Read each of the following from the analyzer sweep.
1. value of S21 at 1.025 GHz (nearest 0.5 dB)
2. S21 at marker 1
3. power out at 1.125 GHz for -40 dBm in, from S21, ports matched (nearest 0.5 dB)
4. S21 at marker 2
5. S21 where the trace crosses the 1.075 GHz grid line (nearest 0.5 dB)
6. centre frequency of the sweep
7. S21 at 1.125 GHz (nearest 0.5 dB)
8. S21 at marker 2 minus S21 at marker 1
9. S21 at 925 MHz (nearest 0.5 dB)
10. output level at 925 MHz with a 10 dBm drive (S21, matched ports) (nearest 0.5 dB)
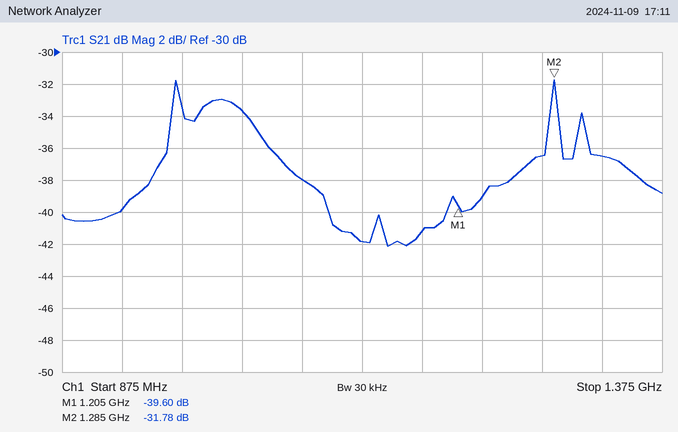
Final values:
-33.5 dB
-39.60 dB
-82.0 dBm
-31.78 dB
-38.0 dB
1.125 GHz
-42.0 dB
7.82 dB
-40.0 dB
-30.0 dBm
